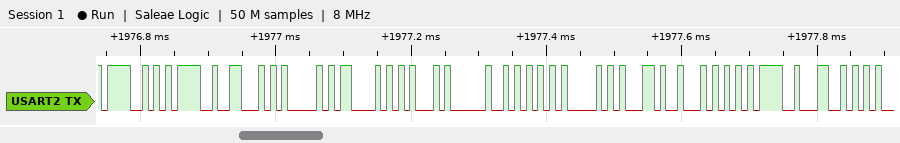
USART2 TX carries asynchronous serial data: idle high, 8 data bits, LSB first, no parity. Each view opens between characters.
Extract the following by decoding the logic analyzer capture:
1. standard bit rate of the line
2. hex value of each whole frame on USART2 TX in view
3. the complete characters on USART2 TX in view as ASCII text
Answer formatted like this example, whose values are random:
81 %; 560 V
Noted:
115200 baud; 4F, 3D, 46, 41, 43, 45, 20, 55, 50, 2C, 54, 3D, 4C; "O=FACE UP,T=L"
